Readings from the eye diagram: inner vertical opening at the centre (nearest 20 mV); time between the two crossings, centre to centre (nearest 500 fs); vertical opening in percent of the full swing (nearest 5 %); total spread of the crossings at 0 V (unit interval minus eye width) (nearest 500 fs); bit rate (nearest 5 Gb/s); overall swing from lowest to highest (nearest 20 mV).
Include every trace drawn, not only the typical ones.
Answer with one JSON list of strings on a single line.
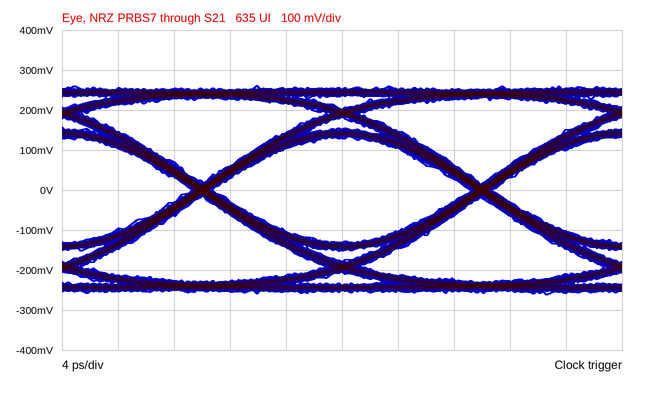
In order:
["260 mV", "20.0 ps", "50 %", "1.5 ps", "50 Gb/s", "520 mV"]
